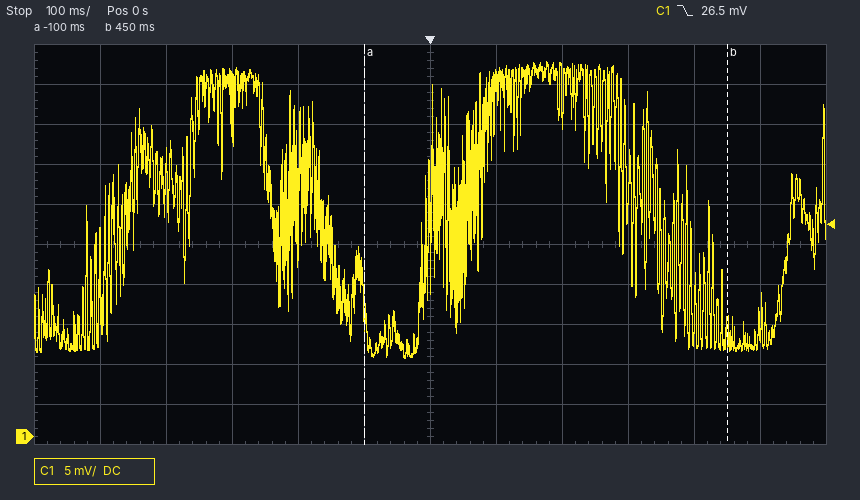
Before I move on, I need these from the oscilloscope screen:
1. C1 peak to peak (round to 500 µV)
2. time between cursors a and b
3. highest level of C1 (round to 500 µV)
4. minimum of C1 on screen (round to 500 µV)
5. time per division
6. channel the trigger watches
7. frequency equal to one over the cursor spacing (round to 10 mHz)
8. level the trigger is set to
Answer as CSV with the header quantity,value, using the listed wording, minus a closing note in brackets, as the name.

quantity,value
C1 peak to peak,37.0 mV
time between cursors a and b,550 ms
highest level of C1,47.0 mV
minimum of C1 on screen,10.0 mV
time per division,100 ms
channel the trigger watches,C1
frequency equal to one over the cursor spacing,1.82 Hz
level the trigger is set to,26.5 mV
